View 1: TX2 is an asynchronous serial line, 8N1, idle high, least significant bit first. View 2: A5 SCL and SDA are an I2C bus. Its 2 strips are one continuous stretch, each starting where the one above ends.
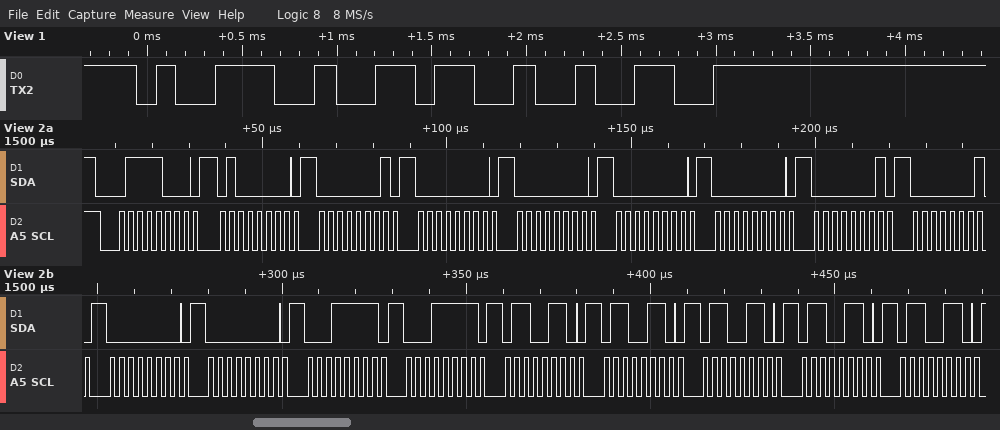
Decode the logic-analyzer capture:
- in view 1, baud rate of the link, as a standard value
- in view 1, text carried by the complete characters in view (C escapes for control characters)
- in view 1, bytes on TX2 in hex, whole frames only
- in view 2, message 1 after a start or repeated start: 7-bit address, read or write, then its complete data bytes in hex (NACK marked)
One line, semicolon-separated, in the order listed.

9600 baud; "962"; 39 36 32; 0x3C write: 40 01 00 00 00 00 01 01 00 00 1F 1F 66 66 66 66 66
